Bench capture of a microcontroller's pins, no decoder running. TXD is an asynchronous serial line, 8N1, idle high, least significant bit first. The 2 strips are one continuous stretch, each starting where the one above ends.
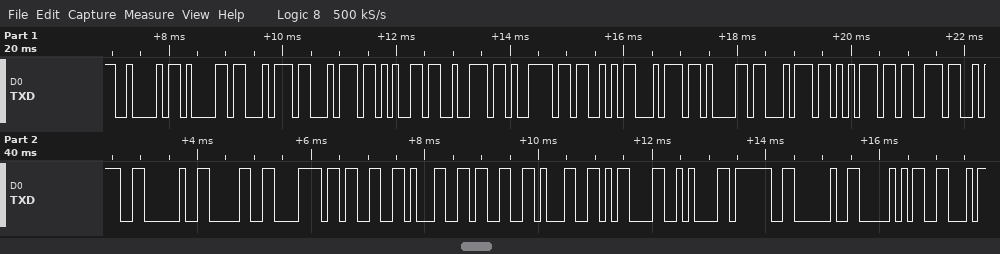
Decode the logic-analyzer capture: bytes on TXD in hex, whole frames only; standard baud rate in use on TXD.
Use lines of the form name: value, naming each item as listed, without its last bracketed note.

bytes on TXD in hex, whole frames only: 42 61 74 74 65 72 79 53 74 61 74 75 73 3A 20 30 78 33 31 33 31 0D 0A 3F 20 50 46
standard baud rate in use on TXD: 9600 baud
